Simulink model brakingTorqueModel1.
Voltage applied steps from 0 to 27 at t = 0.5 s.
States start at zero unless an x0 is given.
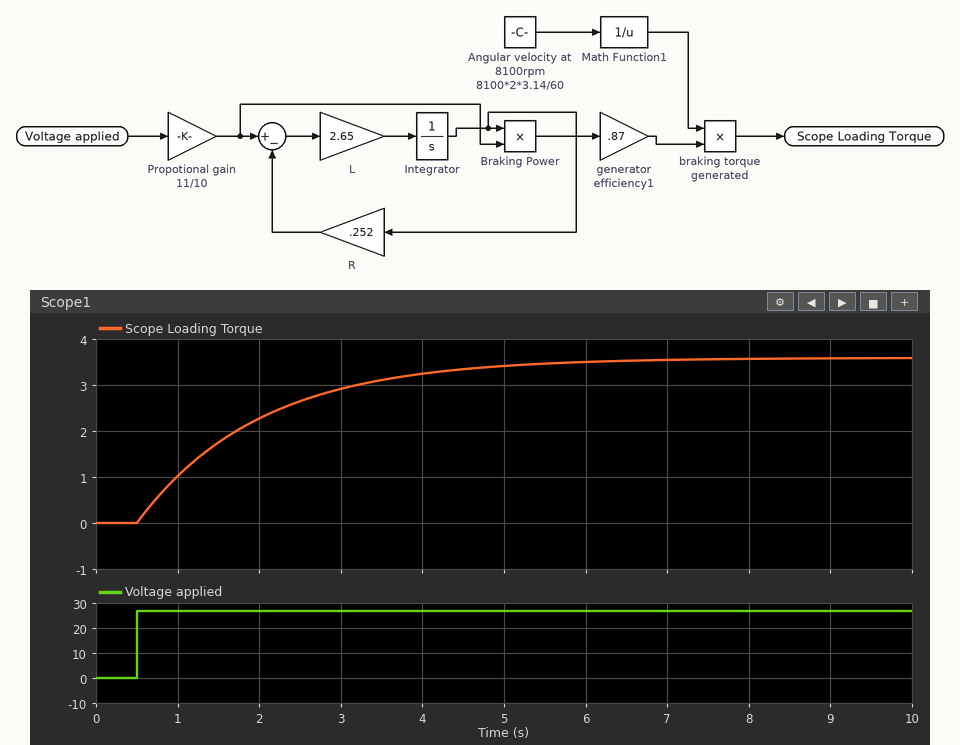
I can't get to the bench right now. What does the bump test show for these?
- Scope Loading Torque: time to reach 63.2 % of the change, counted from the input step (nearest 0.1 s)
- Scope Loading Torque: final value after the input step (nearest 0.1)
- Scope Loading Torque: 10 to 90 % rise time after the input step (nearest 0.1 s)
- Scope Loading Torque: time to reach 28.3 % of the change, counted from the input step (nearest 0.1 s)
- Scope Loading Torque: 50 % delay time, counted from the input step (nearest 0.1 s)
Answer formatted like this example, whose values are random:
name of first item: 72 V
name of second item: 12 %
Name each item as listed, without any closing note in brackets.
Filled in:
Scope Loading Torque: time to reach 63.2 % of the change, counted from the input step: 1.5 s
Scope Loading Torque: final value after the input step: 3.6
Scope Loading Torque: 10 to 90 % rise time after the input step: 3.3 s
Scope Loading Torque: time to reach 28.3 % of the change, counted from the input step: 0.5 s
Scope Loading Torque: 50 % delay time, counted from the input step: 1.0 s
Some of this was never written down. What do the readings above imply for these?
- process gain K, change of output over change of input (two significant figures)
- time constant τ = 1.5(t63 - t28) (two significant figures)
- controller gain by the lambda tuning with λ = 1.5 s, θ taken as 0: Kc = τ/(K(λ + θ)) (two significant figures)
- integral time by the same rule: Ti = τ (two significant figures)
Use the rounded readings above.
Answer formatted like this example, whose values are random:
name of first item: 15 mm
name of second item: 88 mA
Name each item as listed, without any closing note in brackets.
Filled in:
process gain K, change of output over change of input: 0.13
time constant τ = 1.5(t63 - t28): 1.5 s
controller gain by the lambda tuning with λ = 1.5 s, θ taken as 0: Kc = τ/(K(λ + θ)): 7.7
integral time by the same rule: Ti = τ: 1.5 s
